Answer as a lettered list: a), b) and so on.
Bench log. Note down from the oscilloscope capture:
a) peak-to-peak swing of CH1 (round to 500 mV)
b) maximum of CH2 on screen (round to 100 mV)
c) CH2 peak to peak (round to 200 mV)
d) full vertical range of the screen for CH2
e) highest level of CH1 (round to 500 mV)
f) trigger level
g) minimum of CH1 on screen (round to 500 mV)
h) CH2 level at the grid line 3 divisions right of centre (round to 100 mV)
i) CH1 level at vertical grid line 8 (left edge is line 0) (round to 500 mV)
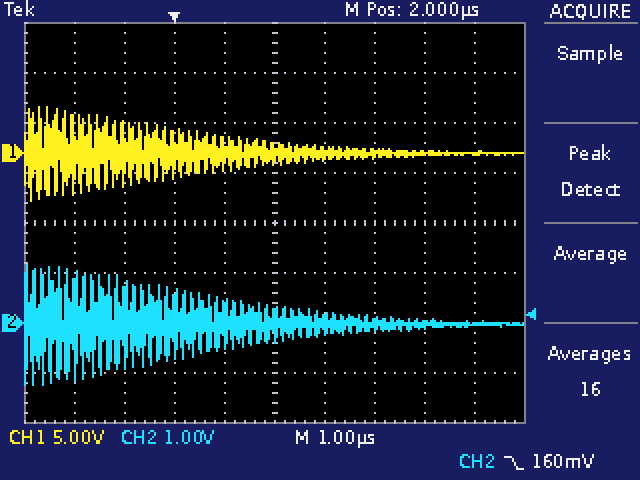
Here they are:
a) 9.5 V
b) 1.2 V
c) 2.4 V
d) 8 V
e) 4.5 V
f) 160 mV
g) -5.0 V
h) 0.0 V
i) 0.0 V
